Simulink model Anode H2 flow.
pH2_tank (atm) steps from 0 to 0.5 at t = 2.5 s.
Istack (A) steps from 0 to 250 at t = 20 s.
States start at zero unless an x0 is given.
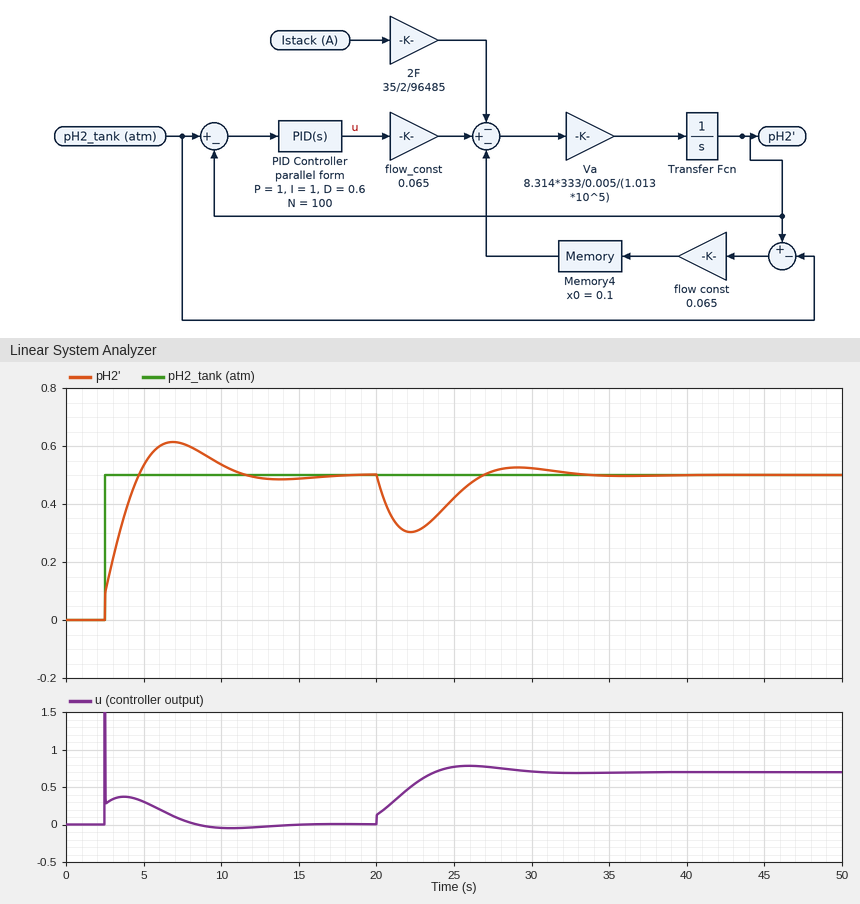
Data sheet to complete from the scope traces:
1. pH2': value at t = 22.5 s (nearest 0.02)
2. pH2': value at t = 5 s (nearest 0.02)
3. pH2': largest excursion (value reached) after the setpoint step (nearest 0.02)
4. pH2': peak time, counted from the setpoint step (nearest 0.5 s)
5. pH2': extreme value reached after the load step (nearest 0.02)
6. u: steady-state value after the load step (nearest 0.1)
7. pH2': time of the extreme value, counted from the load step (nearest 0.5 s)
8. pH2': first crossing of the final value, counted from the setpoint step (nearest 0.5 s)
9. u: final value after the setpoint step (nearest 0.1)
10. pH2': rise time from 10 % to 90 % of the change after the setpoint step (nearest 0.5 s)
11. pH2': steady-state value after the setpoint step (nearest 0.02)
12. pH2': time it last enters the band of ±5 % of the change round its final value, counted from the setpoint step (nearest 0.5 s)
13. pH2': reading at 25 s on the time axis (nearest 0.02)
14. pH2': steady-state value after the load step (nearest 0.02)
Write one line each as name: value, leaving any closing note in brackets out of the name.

pH2': value at t = 22.5 s: 0.30
pH2': value at t = 5 s: 0.54
pH2': largest excursion (value reached) after the setpoint step: 0.62
pH2': peak time, counted from the setpoint step: 4.5 s
pH2': extreme value reached after the load step: 0.30
u: steady-state value after the load step: 0.7
pH2': time of the extreme value, counted from the load step: 2.0 s
pH2': first crossing of the final value, counted from the setpoint step: 2.0 s
u: final value after the setpoint step: 0.0
pH2': rise time from 10 % to 90 % of the change after the setpoint step: 2.0 s
pH2': steady-state value after the setpoint step: 0.50
pH2': time it last enters the band of ±5 % of the change round its final value, counted from the setpoint step: 8.0 s
pH2': reading at 25 s on the time axis: 0.42
pH2': steady-state value after the load step: 0.50
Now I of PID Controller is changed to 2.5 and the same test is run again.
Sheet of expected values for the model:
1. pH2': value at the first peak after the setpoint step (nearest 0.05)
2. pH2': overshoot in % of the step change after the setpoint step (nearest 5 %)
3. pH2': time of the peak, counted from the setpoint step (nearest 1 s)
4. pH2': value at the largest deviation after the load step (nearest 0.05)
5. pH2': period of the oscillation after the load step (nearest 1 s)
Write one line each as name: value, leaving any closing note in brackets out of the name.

pH2': value at the first peak after the setpoint step: 0.65
pH2': overshoot in % of the step change after the setpoint step: 35 %
pH2': time of the peak, counted from the setpoint step: 3 s
pH2': value at the largest deviation after the load step: 0.35
pH2': period of the oscillation after the load step: 8 s
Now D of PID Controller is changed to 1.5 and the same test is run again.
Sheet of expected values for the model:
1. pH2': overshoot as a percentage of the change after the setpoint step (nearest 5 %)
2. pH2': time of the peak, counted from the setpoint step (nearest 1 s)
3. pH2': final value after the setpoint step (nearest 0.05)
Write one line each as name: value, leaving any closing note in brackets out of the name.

pH2': overshoot as a percentage of the change after the setpoint step: 20 %
pH2': time of the peak, counted from the setpoint step: 5 s
pH2': final value after the setpoint step: 0.50
